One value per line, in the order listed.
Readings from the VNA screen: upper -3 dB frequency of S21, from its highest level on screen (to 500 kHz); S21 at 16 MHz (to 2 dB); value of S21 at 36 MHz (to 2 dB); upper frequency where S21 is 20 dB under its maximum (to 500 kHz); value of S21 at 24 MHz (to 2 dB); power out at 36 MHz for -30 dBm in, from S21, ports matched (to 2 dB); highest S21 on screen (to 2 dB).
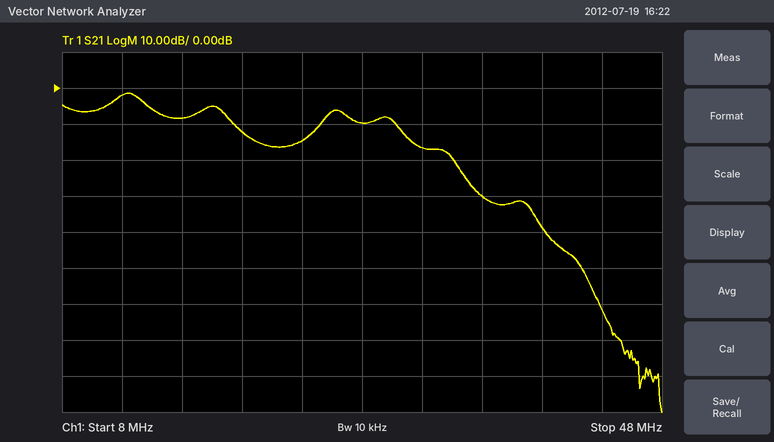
13.5 MHz
-8 dB
-30 dB
34.5 MHz
-14 dB
-60 dBm
-2 dB
